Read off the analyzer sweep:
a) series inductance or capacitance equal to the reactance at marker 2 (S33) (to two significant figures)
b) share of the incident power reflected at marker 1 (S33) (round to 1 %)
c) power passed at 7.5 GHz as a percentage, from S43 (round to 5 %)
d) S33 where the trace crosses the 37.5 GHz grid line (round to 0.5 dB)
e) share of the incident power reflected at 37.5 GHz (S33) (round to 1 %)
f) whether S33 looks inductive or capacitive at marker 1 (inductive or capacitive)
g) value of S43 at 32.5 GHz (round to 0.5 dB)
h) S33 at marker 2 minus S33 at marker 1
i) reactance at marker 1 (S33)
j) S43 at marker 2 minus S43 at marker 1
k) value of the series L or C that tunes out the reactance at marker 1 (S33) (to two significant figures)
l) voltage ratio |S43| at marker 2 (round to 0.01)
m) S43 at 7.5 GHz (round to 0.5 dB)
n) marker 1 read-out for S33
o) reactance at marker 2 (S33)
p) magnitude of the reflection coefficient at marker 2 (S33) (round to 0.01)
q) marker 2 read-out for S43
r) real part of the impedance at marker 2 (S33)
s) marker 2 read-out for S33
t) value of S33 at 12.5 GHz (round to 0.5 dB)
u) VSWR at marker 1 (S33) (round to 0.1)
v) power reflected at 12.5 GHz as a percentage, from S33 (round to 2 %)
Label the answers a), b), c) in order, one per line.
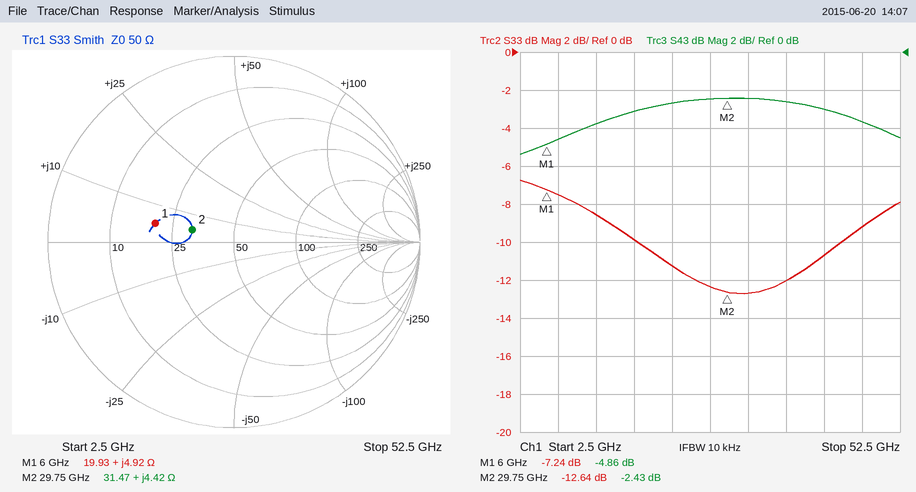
a) 24 pH
b) 19 %
c) 35 %
d) -12.0 dB
e) 6 %
f) inductive
g) -2.5 dB
h) -5.40 dB
i) +4.92 Ω
j) 2.43 dB
k) 5.4 pF
l) 0.76
m) -4.5 dB
n) -7.24 dB
o) +4.42 Ω
p) 0.23
q) -2.43 dB
r) 31.47 Ω
s) -12.64 dB
t) -8.5 dB
u) 2.5
v) 14 %
